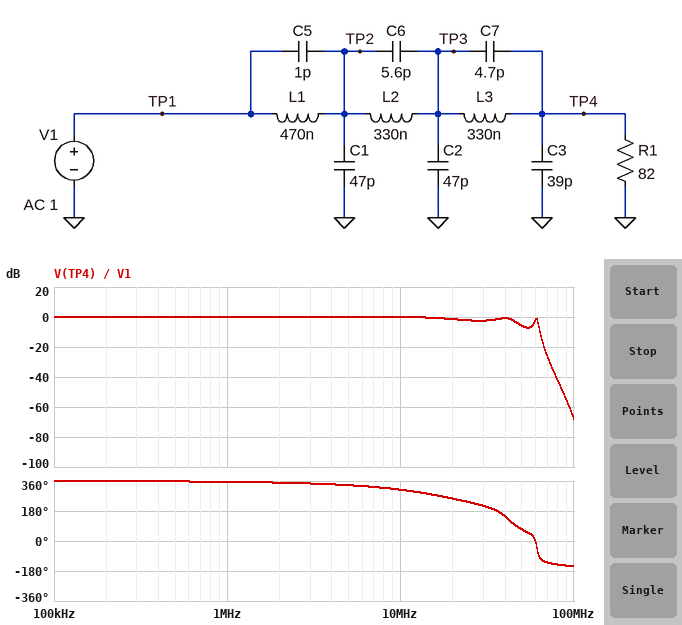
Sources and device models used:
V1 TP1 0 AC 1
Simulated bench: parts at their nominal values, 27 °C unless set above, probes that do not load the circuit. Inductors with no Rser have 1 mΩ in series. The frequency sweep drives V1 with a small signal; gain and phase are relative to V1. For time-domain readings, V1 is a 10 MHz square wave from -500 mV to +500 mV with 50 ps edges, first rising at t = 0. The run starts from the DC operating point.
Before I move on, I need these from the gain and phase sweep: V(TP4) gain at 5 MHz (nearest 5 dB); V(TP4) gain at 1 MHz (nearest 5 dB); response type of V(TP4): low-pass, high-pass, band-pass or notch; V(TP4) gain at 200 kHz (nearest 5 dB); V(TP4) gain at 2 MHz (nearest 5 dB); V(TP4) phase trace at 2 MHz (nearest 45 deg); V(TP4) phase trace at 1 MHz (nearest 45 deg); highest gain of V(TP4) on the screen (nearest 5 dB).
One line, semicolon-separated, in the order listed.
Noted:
0 dB; 0 dB; low-pass; 0 dB; 0 dB; 360 deg; 360 deg; 0 dB
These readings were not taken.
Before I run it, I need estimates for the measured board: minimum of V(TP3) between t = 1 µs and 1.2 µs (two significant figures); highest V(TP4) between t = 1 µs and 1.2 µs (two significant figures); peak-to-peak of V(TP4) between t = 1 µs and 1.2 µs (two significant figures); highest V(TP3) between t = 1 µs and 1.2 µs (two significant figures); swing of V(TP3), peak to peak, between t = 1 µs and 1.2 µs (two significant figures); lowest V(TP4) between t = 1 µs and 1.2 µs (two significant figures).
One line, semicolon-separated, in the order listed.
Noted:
-590 mV; 560 mV; 1.1 V; 590 mV; 1.2 V; -560 mV
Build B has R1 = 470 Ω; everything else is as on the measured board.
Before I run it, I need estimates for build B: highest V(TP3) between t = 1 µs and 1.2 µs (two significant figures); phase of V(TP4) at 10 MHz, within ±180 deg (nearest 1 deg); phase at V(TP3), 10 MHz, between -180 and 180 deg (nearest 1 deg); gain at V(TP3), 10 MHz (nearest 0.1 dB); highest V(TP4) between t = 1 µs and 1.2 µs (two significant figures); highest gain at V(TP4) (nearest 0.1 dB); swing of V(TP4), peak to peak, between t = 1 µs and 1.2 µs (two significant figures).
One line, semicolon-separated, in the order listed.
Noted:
1.0 V; -13 deg; -10 deg; 3.6 dB; 1.3 V; 14.4 dB; 2.7 V
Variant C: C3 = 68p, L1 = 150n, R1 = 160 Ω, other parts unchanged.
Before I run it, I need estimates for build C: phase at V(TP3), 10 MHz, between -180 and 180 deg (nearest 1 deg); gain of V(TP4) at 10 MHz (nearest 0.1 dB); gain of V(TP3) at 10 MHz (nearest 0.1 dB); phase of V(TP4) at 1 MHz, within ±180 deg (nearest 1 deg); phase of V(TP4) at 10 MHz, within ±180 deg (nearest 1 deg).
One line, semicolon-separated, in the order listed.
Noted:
-16 deg; 2.6 dB; 1.9 dB; -2 deg; -24 deg
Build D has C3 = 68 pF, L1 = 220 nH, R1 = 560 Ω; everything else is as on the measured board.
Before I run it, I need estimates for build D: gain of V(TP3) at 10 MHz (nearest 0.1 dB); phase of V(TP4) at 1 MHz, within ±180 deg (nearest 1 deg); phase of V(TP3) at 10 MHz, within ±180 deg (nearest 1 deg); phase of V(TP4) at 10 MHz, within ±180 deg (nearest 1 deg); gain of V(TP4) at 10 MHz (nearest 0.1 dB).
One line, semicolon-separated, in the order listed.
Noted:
3.0 dB; -1 deg; -6 deg; -8 deg; 3.8 dB
